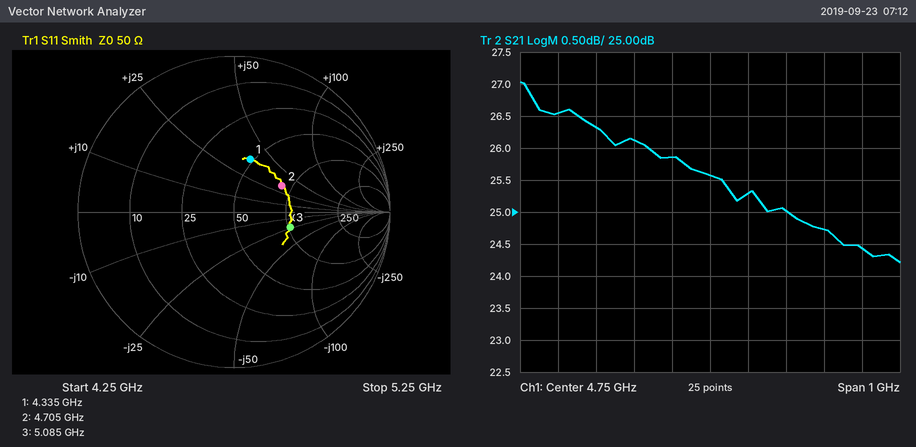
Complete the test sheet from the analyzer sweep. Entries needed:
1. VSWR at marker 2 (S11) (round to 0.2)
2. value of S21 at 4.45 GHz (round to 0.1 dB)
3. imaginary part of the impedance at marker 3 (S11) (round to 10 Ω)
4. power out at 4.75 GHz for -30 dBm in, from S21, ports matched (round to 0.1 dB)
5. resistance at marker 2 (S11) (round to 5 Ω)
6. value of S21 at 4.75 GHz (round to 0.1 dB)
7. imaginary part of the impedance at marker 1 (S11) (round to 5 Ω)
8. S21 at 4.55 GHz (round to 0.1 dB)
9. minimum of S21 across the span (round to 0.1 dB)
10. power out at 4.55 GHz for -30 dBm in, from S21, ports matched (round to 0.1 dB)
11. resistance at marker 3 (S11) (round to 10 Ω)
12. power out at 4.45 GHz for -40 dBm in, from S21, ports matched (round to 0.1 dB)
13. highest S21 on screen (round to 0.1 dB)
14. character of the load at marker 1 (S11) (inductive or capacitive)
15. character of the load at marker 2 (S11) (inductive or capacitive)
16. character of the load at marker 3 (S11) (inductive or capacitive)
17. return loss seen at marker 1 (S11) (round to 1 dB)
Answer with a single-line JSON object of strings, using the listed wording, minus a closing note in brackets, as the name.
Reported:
{"VSWR at marker 2 (S11)": "2.0", "value of S21 at 4.45 GHz": "26.3 dB", "imaginary part of the impedance at marker 3 (S11)": "-20 Ω", "power out at 4.75 GHz for -30 dBm in, from S21, ports matched": "-4.4 dBm", "resistance at marker 2 (S11)": "85 Ω", "value of S21 at 4.75 GHz": "25.6 dB", "imaginary part of the impedance at marker 1 (S11)": "+35 Ω", "S21 at 4.55 GHz": "26.1 dB", "minimum of S21 across the span": "24.2 dB", "power out at 4.55 GHz for -30 dBm in, from S21, ports matched": "-3.9 dBm", "resistance at marker 3 (S11)": "100 Ω", "power out at 4.45 GHz for -40 dBm in, from S21, ports matched": "-13.7 dBm", "highest S21 on screen": "27.0 dB", "character of the load at marker 1 (S11)": "inductive", "character of the load at marker 2 (S11)": "inductive", "character of the load at marker 3 (S11)": "capacitive", "return loss seen at marker 1 (S11)": "9 dB"}
